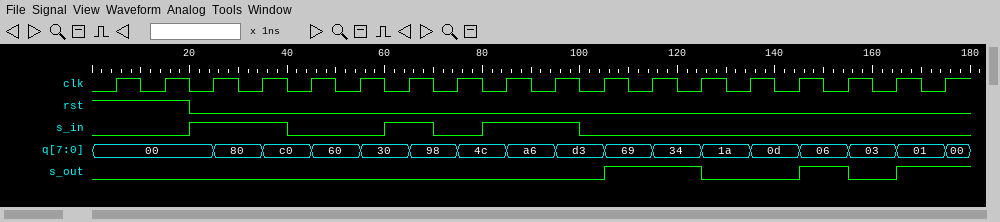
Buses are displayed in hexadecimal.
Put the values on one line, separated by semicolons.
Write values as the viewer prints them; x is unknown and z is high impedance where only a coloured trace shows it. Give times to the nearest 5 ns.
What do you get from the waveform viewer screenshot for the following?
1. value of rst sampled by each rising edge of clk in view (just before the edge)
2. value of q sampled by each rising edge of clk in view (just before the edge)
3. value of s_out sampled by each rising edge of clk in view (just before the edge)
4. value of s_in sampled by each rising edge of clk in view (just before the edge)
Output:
1 1 0 0 0 0 0 0 0 0 0 0 0 0 0 0 0 0; 00, 00, 00, 80, c0, 60, 30, 98, 4c, a6, d3, 69, 34, 1a, 0d, 06, 03, 01; 0 0 0 0 0 0 0 0 0 0 0 1 1 0 0 1 0 1; 0 0 1 1 0 0 1 0 1 1 0 0 0 0 0 0 0 0
